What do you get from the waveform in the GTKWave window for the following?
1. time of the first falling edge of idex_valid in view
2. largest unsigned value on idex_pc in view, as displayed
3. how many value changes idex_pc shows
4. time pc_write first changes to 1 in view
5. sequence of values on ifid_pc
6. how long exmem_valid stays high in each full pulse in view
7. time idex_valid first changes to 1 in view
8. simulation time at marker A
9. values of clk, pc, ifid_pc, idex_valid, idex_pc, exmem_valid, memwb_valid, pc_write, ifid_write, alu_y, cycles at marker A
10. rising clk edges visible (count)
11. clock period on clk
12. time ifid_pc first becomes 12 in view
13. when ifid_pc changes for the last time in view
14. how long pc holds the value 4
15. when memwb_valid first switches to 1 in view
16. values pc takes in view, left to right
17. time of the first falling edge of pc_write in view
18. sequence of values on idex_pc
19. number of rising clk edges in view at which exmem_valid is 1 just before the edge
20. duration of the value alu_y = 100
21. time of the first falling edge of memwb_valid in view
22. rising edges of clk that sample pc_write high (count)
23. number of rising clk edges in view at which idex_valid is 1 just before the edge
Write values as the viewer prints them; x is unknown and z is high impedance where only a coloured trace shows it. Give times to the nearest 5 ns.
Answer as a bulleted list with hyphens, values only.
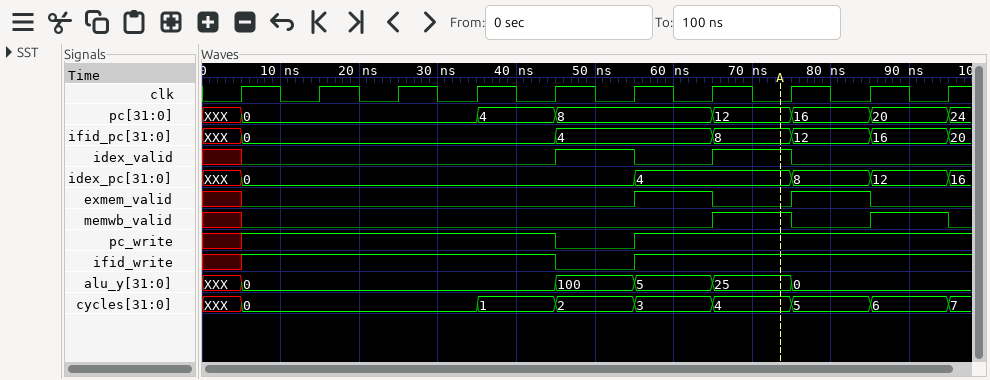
- 55 ns
- 16
- 5
- 5 ns
- XXX, 0, 4, 8, 12, 16, 20
- 10 ns, 10 ns
- 45 ns
- 75 ns
- clk=0, pc=12, ifid_pc=8, idex_valid=1, idex_pc=4, exmem_valid=0, memwb_valid=1, pc_write=1, ifid_write=1, alu_y=25, cycles=4
- 10
- 10 ns
- 75 ns
- 95 ns
- 10 ns
- 65 ns
- XXX, 0, 4, 8, 12, 16, 20, 24
- 45 ns
- XXX, 0, 4, 8, 12, 16
- 2
- 10 ns
- 75 ns
- 8
- 2
